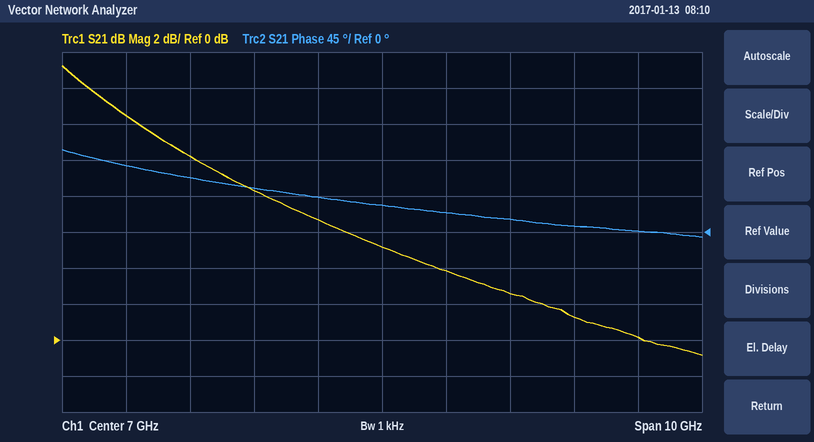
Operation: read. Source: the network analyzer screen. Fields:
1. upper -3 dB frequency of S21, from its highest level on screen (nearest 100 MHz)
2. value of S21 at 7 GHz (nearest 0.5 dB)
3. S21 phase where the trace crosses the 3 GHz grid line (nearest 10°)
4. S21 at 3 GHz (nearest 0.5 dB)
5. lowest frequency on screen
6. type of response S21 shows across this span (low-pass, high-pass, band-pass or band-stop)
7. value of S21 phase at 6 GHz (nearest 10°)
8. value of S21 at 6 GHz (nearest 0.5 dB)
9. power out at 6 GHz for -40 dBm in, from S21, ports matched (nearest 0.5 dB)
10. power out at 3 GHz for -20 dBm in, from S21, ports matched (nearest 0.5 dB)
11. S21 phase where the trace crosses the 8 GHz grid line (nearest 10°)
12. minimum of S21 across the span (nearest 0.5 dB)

3.1 GHz
5.0 dB
80°
12.5 dB
2 GHz
low-pass
40°
6.5 dB
-33.5 dBm
-7.5 dBm
20°
-1.0 dB
